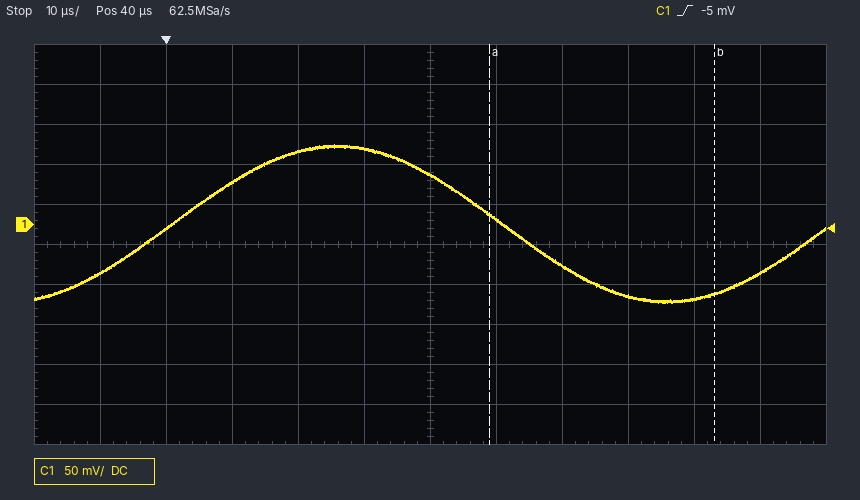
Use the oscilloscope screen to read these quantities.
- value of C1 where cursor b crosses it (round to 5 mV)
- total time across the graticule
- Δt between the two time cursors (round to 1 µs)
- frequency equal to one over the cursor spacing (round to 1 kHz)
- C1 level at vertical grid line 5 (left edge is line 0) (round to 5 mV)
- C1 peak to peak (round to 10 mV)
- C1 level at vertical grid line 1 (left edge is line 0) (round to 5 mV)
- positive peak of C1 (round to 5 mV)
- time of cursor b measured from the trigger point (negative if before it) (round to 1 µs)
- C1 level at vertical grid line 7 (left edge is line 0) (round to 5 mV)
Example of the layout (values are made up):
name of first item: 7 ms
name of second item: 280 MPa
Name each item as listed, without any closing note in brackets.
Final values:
value of C1 where cursor b crosses it: -85 mV
total time across the graticule: 120 µs
Δt between the two time cursors: 34 µs
frequency equal to one over the cursor spacing: 29 kHz
C1 level at vertical grid line 5 (left edge is line 0): 95 mV
C1 peak to peak: 200 mV
C1 level at vertical grid line 1 (left edge is line 0): -60 mV
positive peak of C1: 100 mV
time of cursor b measured from the trigger point (negative if before it): +83 µs
C1 level at vertical grid line 7 (left edge is line 0): 5 mV
